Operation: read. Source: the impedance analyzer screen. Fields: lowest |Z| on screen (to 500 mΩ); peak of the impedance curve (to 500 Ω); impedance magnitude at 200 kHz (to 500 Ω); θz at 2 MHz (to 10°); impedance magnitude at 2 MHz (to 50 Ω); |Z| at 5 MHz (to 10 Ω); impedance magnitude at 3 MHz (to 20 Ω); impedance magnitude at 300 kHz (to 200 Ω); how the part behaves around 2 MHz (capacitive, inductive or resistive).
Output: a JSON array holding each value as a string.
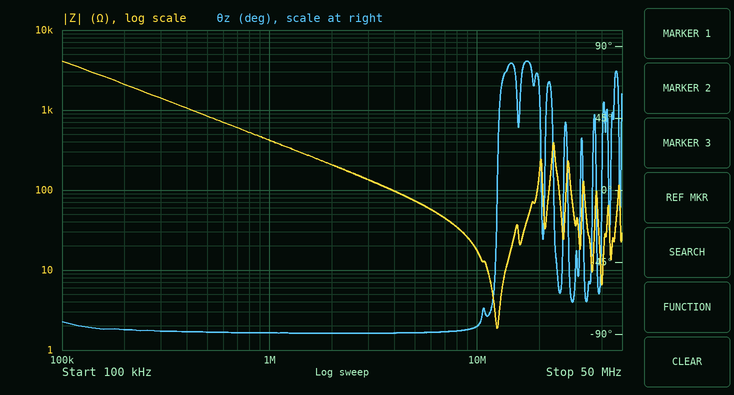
["2.0 Ω", "4.0 kΩ", "2.0 kΩ", "-90°", "200 Ω", "70 Ω", "140 Ω", "1.4 kΩ", "capacitive"]
